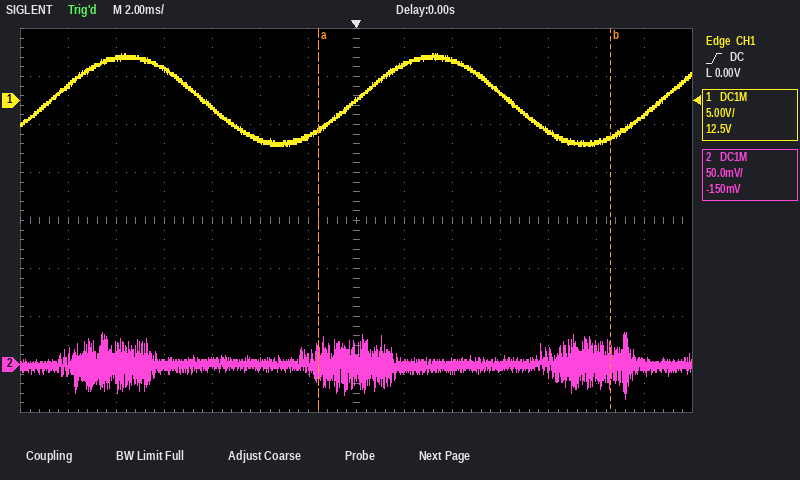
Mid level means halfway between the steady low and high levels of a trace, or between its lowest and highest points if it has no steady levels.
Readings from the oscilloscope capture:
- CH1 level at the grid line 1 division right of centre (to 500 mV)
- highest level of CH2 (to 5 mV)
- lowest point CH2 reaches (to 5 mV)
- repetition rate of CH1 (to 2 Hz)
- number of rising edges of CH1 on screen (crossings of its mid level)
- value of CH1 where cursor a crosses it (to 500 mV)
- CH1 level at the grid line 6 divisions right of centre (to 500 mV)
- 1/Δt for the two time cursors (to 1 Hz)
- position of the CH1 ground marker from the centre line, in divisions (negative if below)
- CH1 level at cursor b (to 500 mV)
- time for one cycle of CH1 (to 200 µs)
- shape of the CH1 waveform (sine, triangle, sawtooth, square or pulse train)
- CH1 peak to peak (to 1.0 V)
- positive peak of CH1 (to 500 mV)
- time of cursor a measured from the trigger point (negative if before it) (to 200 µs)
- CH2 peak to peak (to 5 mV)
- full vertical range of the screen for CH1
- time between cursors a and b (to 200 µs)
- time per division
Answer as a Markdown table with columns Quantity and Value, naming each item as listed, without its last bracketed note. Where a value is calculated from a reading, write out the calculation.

| Quantity | Value |
|---|---|
| CH1 level at the grid line 1 division right of centre | 3.5 V |
| highest level of CH2 | 35 mV |
| lowest point CH2 reaches | -35 mV |
| repetition rate of CH1 | 1 / 12.8 ms ≈ 78 Hz |
| number of rising edges of CH1 on screen | 3 |
| value of CH1 where cursor a crosses it | -3.0 V |
| CH1 level at the grid line 6 divisions right of centre | -1.5 V |
| 1/Δt for the two time cursors | 1 / 12.2 ms ≈ 82 Hz |
| position of the CH1 ground marker from the centre line, in divisions | +2.5 div |
| CH1 level at cursor b | -4.0 V |
| time for one cycle of CH1 | 12.8 ms |
| shape of the CH1 waveform | sine |
| CH1 peak to peak | 10.0 V |
| positive peak of CH1 | 5.0 V |
| time of cursor a measured from the trigger point (negative if before it) | -1.6 ms |
| CH2 peak to peak | 35 mV − (-35 mV) = 70 mV |
| full vertical range of the screen for CH1 | 40 V |
| time between cursors a and b | 12.2 ms |
| time per division | 2 ms |
